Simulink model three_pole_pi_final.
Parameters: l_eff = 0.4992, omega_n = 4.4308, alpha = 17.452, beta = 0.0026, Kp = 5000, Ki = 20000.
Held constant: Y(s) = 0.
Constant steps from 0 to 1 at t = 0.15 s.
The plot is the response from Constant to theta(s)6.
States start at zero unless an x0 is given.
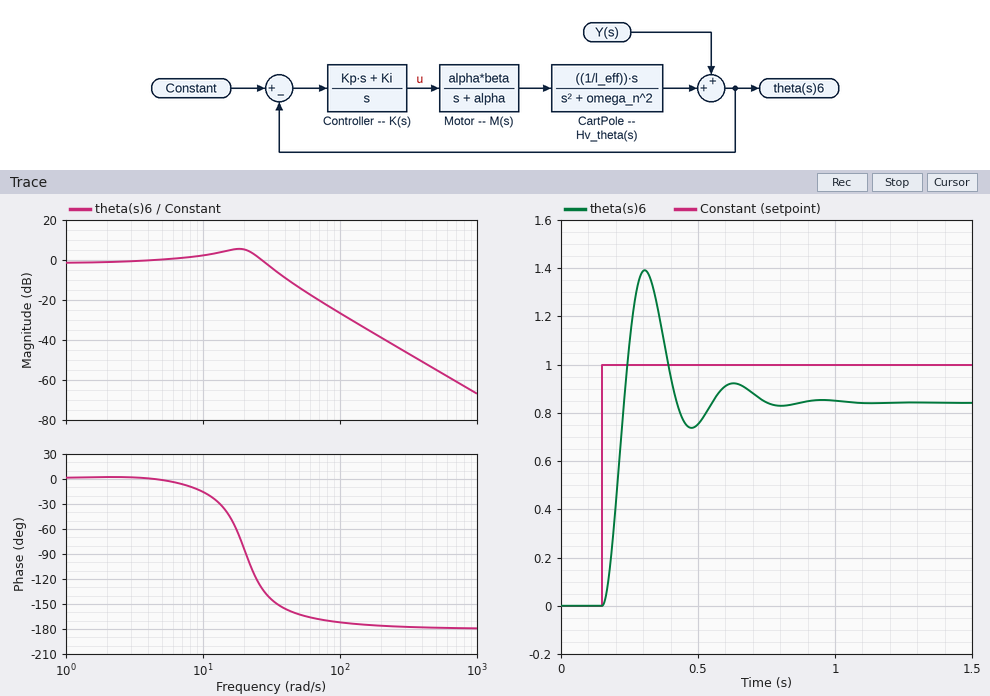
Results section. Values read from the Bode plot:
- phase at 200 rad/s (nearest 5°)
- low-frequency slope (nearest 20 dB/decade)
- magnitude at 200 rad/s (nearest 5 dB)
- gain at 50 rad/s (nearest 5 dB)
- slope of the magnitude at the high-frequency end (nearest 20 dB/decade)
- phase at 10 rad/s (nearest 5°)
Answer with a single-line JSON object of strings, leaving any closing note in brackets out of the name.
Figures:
{"phase at 200 rad/s": "-175°", "low-frequency slope": "0 dB/decade", "magnitude at 200 rad/s": "-40 dB", "gain at 50 rad/s": "-15 dB", "slope of the magnitude at the high-frequency end": "-40 dB/decade", "phase at 10 rad/s": "-15°"}
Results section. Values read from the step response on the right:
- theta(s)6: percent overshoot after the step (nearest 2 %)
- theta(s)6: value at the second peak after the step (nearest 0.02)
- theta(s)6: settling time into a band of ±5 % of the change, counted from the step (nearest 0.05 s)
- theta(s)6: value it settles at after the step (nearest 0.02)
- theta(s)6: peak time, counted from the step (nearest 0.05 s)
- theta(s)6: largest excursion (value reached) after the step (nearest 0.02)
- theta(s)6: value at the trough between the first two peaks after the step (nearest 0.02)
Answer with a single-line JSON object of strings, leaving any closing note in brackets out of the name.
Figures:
{"theta(s)6: percent overshoot after the step": "66 %", "theta(s)6: value at the second peak after the step": "0.92", "theta(s)6: settling time into a band of ±5 % of the change, counted from the step": "0.55 s", "theta(s)6: value it settles at after the step": "0.84", "theta(s)6: peak time, counted from the step": "0.15 s", "theta(s)6: largest excursion (value reached) after the step": "1.40", "theta(s)6: value at the trough between the first two peaks after the step": "0.74"}
